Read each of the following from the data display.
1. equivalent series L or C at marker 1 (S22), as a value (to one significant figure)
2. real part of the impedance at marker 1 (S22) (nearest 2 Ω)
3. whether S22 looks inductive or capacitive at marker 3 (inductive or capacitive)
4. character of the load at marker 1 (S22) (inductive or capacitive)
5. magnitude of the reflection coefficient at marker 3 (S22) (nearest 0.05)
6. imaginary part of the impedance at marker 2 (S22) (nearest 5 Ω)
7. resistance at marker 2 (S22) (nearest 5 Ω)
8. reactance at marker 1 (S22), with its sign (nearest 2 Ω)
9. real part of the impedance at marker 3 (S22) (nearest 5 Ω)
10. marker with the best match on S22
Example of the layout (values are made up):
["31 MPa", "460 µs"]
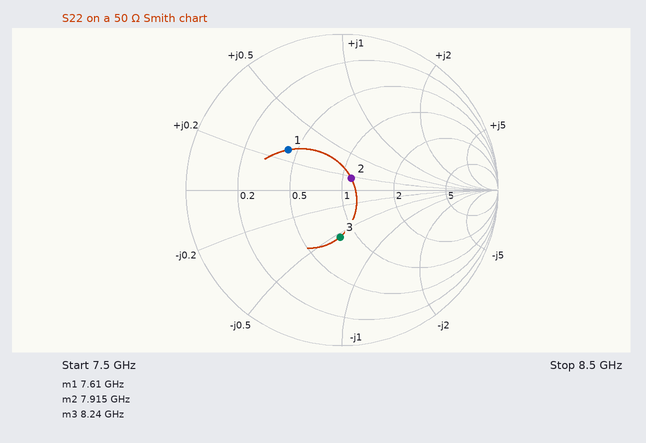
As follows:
["300 pH", "22 Ω", "capacitive", "inductive", "0.30", "+10 Ω", "55 Ω", "+14 Ω", "40 Ω", "marker 2"]
